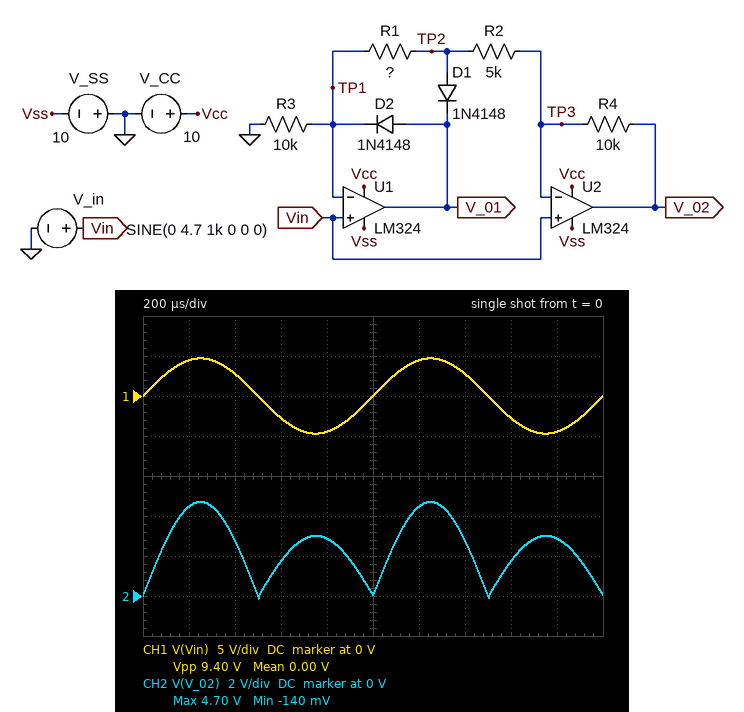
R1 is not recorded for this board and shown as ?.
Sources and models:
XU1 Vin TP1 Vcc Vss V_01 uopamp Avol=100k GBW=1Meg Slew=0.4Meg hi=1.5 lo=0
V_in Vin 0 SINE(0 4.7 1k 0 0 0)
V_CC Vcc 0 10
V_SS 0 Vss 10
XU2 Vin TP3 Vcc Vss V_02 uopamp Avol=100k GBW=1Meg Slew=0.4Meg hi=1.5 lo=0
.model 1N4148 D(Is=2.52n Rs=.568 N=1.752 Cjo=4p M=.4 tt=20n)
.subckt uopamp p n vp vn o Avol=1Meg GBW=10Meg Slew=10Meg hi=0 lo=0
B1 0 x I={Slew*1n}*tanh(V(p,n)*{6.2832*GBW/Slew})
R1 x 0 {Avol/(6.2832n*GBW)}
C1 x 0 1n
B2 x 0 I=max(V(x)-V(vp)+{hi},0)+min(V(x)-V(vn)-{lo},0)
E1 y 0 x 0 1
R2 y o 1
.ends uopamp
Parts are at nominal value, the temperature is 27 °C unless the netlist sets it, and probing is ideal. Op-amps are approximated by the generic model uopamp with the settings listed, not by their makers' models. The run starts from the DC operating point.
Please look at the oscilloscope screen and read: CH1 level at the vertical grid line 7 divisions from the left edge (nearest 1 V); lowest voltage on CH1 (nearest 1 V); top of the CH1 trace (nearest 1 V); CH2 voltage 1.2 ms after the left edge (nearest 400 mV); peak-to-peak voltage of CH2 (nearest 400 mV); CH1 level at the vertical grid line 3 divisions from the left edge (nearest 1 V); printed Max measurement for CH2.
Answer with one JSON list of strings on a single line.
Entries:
["3 V", "-5 V", "5 V", "4.4 V", "4.8 V", "-3 V", "4.70 V"]
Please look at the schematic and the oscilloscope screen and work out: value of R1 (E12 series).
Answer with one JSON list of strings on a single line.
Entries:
["8.2 kΩ"]
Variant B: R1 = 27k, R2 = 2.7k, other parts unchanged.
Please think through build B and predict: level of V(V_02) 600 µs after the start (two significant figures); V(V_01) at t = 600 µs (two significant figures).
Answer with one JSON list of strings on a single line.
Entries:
["8.5 V", "-10 V"]
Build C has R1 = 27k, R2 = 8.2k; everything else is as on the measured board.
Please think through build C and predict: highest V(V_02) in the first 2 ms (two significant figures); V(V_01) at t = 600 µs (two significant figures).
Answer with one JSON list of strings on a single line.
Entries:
["5.8 V", "-10 V"]
